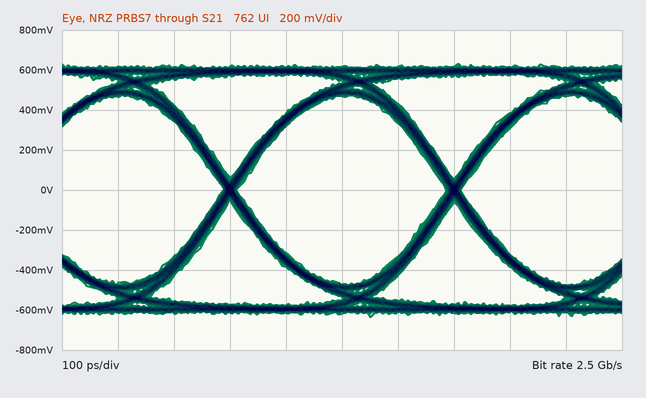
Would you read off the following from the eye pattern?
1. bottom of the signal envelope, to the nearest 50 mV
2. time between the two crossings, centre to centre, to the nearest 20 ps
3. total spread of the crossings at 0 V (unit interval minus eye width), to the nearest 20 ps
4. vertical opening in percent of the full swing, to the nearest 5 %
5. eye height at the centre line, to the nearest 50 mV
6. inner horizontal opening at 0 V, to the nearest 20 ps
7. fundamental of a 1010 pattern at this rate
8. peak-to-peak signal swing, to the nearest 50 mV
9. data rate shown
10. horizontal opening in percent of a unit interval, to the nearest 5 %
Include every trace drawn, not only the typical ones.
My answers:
-650 mV
400 ps
20 ps
75 %
950 mV
380 ps
1.25 GHz
1.25 V
2.5 Gb/s
95 %
